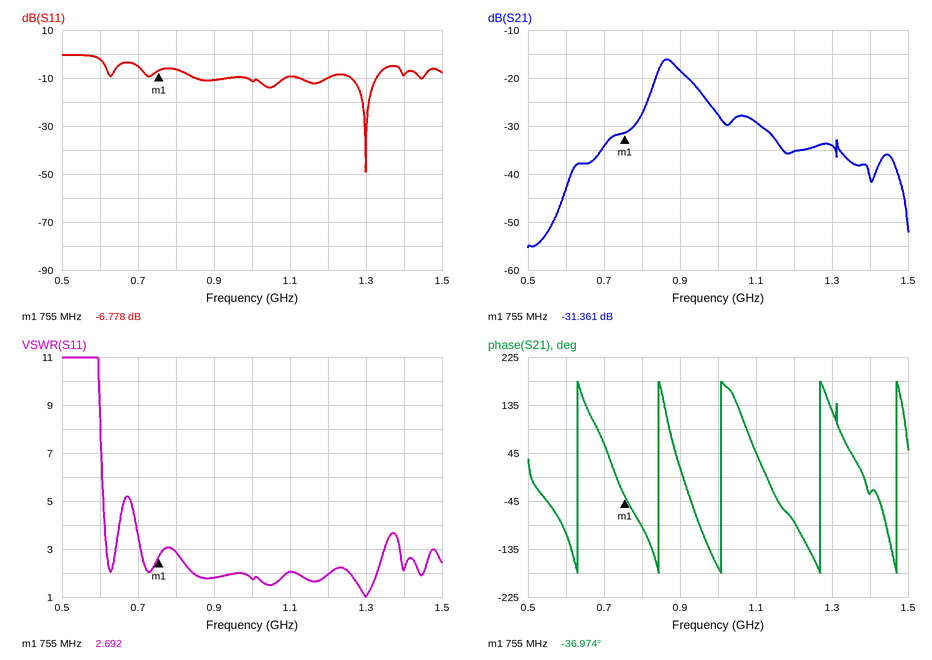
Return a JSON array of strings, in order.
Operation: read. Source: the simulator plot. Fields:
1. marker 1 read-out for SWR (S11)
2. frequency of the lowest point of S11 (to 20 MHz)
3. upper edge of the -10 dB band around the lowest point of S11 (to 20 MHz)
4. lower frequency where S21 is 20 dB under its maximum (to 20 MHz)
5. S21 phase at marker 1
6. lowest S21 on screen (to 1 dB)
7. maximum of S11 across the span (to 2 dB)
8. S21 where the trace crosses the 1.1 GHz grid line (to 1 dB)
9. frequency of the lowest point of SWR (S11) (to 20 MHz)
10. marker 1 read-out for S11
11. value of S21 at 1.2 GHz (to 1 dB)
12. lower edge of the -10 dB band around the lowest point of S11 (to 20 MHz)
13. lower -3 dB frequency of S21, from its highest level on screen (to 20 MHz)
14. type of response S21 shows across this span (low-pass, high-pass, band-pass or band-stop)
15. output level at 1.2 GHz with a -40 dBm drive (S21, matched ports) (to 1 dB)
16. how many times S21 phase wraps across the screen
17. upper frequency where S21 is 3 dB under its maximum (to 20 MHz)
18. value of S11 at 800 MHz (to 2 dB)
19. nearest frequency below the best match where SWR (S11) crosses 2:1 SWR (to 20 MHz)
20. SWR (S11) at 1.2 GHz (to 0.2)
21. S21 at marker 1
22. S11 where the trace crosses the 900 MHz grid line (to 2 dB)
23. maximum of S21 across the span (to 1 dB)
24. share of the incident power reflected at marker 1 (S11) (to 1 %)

["2.692", "1.30 GHz", "1.32 GHz", "680 MHz", "-36.974°", "-55 dB", "0 dB", "-29 dB", "1.30 GHz", "-6.778 dB", "-35 dB", "1.26 GHz", "840 MHz", "band-pass", "-75 dBm", "5", "900 MHz", "-6 dB", "1.26 GHz", "2.0", "-31.361 dB", "-10 dB", "-16 dB", "21 %"]
